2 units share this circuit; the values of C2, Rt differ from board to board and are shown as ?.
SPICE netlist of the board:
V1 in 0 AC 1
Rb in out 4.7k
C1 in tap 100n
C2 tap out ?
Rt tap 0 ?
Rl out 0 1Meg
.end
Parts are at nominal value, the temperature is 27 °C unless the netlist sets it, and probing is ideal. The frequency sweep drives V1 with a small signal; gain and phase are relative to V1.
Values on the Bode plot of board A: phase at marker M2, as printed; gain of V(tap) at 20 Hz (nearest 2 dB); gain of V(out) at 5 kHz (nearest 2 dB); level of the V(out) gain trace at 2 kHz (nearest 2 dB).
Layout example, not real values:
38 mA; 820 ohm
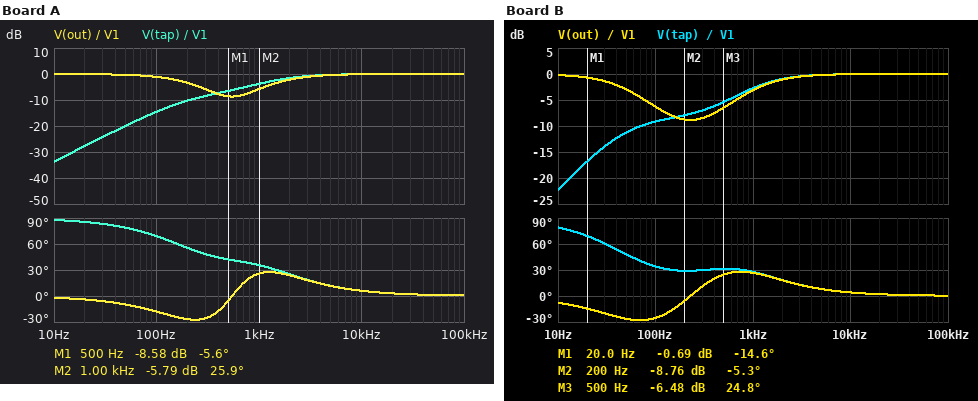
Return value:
25.9 deg; -28 dB; 0 dB; -2 dB
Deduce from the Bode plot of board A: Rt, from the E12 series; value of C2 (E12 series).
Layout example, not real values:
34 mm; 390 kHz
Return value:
1.5 kΩ; 120 nF
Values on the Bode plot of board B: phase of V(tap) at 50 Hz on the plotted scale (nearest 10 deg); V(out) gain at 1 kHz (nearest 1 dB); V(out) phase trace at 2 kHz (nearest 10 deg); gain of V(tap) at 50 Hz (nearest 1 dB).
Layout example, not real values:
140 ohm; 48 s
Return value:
50 deg; -3 dB; 20 deg; -11 dB
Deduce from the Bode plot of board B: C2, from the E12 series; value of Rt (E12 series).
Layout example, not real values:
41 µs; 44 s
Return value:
470 nF; 2.2 kΩ
